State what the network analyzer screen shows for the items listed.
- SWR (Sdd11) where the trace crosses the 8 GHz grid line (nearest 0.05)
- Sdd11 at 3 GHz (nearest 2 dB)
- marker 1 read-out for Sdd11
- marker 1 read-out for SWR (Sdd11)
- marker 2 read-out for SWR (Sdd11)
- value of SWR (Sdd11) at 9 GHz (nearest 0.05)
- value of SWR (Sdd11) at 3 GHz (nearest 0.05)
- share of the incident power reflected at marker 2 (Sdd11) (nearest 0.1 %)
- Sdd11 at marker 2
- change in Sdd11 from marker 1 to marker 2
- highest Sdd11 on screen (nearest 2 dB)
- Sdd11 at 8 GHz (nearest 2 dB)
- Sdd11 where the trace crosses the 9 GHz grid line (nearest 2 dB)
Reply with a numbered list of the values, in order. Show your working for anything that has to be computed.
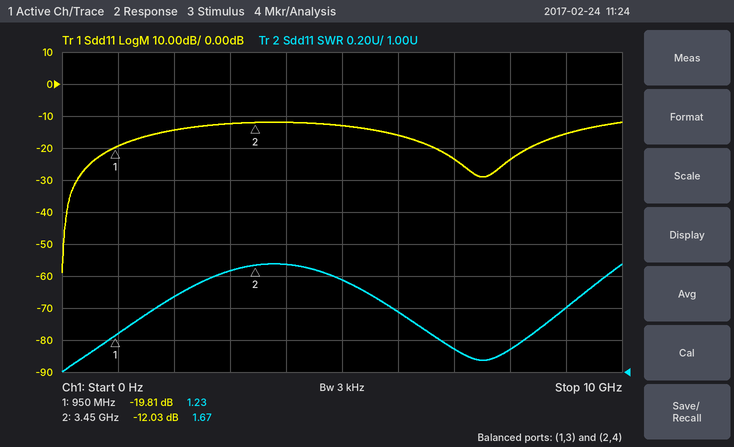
1. 1.15
2. -12 dB
3. -19.81 dB
4. 1.23
5. 1.67
6. 1.40
7. 1.65
8. 10^(-12.03/10) ≈ 6.3 %
9. -12.03 dB
10. -12.03 − (-19.81) = 7.78 dB
11. -12 dB
12. -24 dB
13. -16 dB
